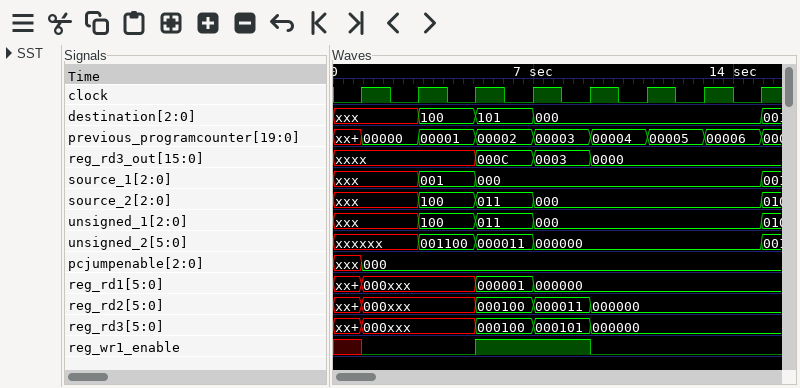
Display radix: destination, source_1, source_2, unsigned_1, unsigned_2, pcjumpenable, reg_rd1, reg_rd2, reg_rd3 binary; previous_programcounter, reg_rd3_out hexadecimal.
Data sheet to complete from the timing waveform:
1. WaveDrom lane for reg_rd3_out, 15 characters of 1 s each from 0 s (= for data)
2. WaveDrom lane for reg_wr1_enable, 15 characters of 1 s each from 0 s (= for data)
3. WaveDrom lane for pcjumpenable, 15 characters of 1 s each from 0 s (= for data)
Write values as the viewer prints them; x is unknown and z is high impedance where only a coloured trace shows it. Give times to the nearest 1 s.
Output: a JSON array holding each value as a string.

["{name: 'reg_rd3_out', wave: 'x....=.=.=.....', data: '000C 0003 0000'}", "{name: 'reg_wr1_enable', wave: 'x0...1...0.....'}", "{name: 'pcjumpenable', wave: 'x=.............', data: '000'}"]
